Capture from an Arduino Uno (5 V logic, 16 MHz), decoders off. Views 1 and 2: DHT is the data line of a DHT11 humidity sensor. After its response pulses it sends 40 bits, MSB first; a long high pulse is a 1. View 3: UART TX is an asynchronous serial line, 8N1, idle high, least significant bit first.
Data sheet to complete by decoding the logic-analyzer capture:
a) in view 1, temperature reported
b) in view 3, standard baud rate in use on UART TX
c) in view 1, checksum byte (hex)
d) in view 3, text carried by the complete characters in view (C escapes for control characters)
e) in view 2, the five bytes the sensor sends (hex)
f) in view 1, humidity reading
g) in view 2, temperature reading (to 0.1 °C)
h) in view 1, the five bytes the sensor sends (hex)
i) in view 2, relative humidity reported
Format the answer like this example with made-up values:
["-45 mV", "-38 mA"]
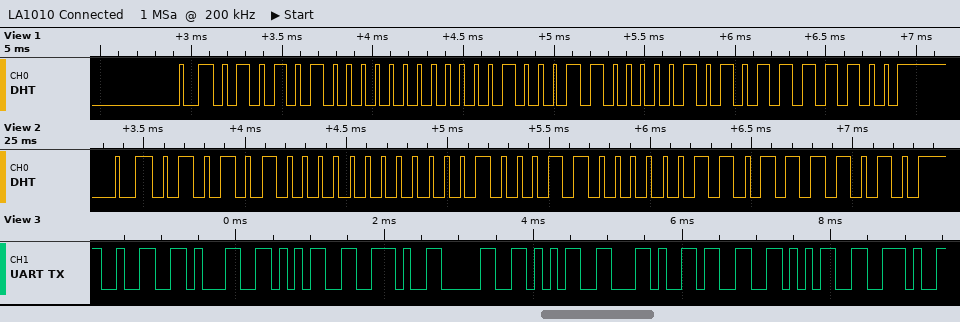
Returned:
["35.5 °C", "9600 baud", "0x7C", "\"215.05,35.\"", "54 00 23 03 7A", "84 %", "35.3 °C", "54 00 23 05 7C", "84 %"]
